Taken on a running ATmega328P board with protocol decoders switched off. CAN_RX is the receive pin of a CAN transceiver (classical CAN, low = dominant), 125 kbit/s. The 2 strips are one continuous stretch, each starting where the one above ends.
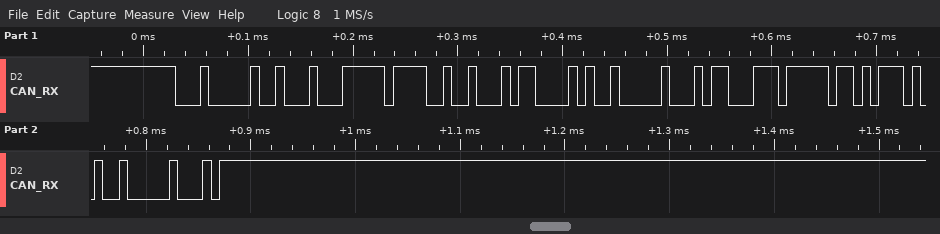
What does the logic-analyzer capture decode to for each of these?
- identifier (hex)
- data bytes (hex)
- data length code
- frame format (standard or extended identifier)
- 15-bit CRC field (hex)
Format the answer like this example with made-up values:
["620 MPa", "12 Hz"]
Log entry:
["0x101", "FF 92 2C 29 00 B1 DF D7", "8", "standard", "0x2900"]
